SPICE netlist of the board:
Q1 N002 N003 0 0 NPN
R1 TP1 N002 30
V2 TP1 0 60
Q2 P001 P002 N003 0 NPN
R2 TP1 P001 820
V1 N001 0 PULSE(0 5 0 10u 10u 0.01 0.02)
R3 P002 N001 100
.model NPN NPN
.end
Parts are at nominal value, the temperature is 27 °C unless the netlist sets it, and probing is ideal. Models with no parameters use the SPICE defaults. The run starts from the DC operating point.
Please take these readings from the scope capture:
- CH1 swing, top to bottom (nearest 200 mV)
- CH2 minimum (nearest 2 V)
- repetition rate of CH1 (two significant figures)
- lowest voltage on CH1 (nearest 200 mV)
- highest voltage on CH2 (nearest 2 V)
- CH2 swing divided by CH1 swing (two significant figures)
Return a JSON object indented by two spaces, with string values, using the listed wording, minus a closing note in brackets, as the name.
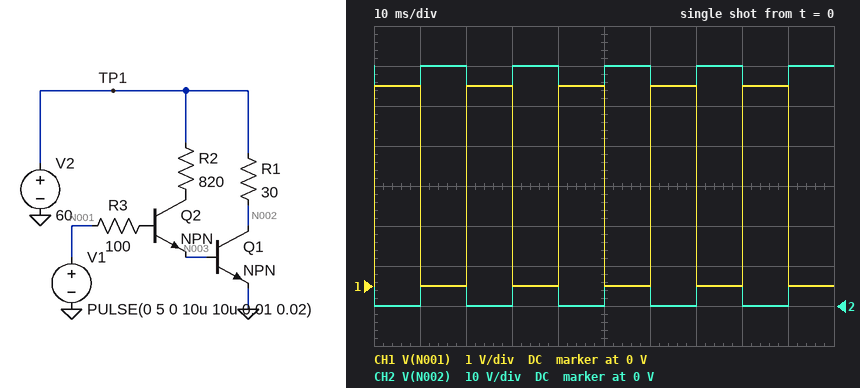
{
  "CH1 swing, top to bottom": "5.0 V",
  "CH2 minimum": "0 V",
  "repetition rate of CH1": "50 Hz",
  "lowest voltage on CH1": "0 V",
  "highest voltage on CH2": "60 V",
  "CH2 swing divided by CH1 swing": "12"
}
